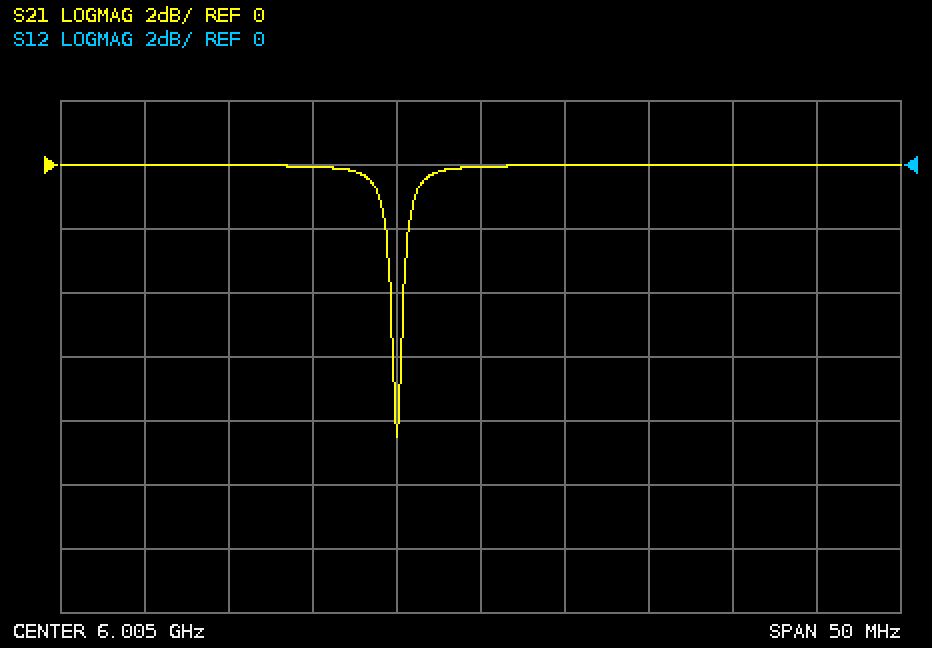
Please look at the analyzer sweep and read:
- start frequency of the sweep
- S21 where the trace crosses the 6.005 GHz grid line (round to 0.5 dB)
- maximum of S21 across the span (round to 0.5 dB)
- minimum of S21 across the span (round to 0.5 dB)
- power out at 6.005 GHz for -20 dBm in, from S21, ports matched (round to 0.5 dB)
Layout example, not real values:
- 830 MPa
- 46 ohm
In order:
- 5.98 GHz
- 0.0 dB
- 0.0 dB
- -8.5 dB
- -20.0 dBm
